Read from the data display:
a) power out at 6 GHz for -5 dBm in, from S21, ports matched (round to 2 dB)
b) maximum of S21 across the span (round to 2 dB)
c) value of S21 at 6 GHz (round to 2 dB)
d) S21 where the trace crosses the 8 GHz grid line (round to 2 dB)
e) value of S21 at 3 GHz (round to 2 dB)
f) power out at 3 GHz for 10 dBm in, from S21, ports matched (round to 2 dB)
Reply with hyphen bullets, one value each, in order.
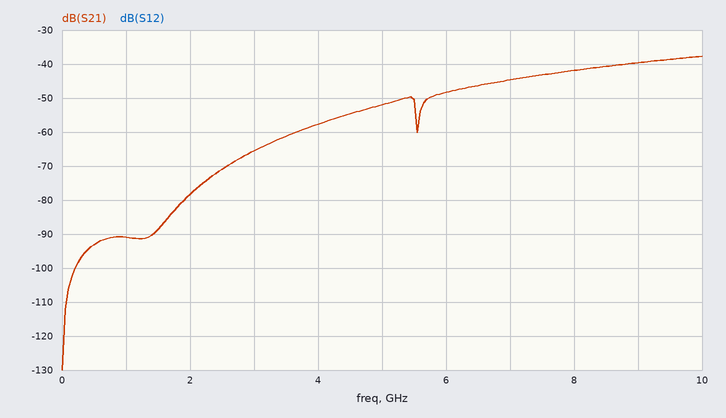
- -54 dBm
- -38 dB
- -48 dB
- -42 dB
- -66 dB
- -56 dBm
